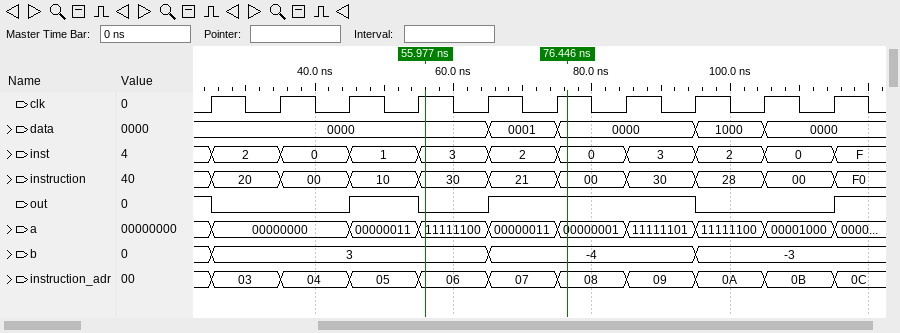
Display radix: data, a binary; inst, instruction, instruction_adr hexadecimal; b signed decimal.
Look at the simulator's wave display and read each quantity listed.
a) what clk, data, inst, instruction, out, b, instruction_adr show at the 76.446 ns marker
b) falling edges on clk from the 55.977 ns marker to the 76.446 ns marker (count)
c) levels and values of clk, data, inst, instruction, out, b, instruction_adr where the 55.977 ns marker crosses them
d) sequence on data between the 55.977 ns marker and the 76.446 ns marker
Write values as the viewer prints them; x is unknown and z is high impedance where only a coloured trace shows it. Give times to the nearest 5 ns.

clk=1, data=0000, inst=0, instruction=00, out=1, b=-4, instruction_adr=08
2
clk=1, data=0000, inst=3, instruction=30, out=0, b=3, instruction_adr=06
0000, 0001, 0000
